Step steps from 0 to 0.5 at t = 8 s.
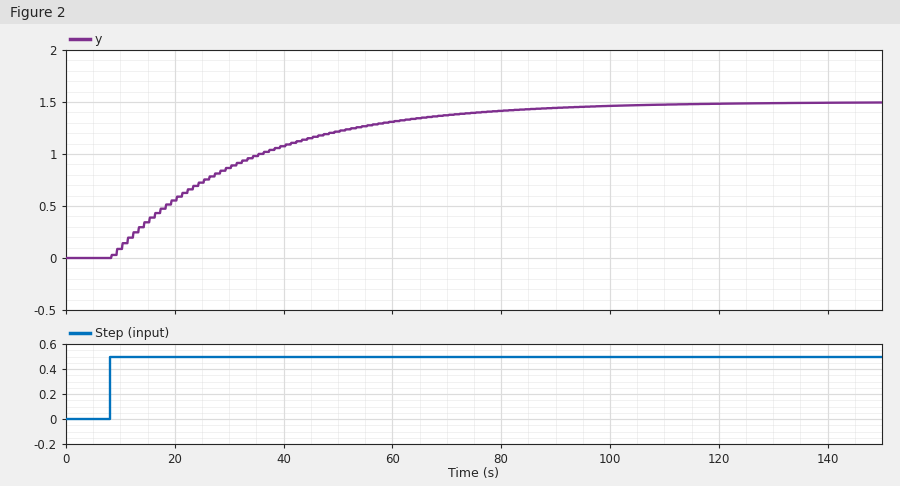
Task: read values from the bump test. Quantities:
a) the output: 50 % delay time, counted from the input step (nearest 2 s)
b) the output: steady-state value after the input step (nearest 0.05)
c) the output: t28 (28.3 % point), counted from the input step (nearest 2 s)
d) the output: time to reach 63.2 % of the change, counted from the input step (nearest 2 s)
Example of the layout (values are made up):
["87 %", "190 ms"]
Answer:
["18 s", "1.50", "8 s", "26 s"]
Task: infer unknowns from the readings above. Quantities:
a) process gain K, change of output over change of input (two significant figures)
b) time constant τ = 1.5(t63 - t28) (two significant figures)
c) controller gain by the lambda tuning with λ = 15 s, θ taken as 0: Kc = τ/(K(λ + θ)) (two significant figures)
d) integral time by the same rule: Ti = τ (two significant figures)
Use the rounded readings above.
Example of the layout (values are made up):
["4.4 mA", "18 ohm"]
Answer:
["3.0", "27 s", "0.60", "27 s"]
